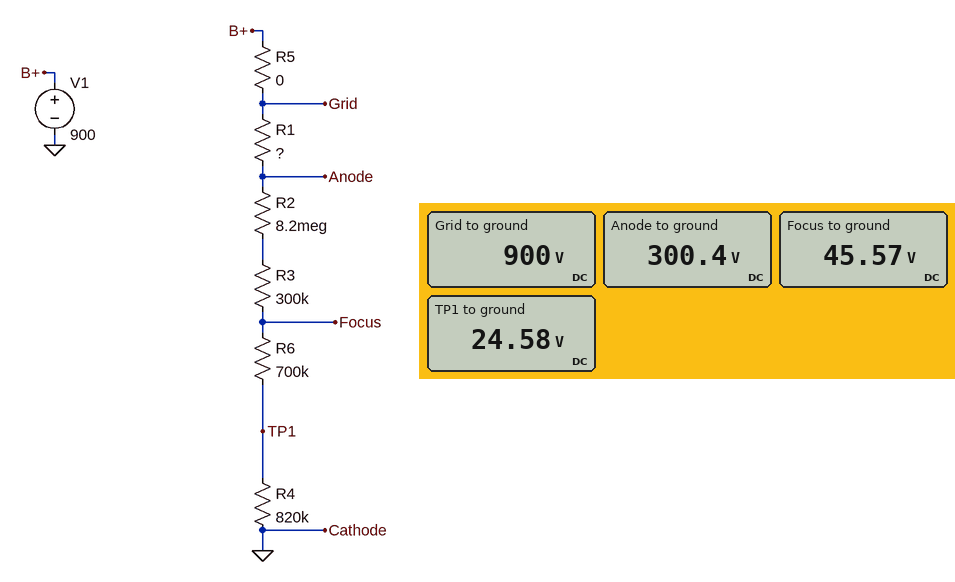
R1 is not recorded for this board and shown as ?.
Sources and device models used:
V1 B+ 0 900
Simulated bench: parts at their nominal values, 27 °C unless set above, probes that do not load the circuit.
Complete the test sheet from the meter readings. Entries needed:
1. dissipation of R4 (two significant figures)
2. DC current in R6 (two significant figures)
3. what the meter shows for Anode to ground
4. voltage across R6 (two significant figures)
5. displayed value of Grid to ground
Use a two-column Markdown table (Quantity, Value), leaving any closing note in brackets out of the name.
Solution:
| Quantity | Value |
|---|---|
| dissipation of R4 | 740 µW |
| DC current in R6 | 30 µA |
| what the meter shows for Anode to ground | 300.4 V |
| voltage across R6 | 21 V |
| displayed value of Grid to ground | 900 V |
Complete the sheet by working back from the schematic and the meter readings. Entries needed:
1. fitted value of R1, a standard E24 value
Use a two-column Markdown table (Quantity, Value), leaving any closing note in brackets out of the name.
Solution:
| Quantity | Value |
|---|---|
| fitted value of R1, a standard E24 value | 20 MΩ |
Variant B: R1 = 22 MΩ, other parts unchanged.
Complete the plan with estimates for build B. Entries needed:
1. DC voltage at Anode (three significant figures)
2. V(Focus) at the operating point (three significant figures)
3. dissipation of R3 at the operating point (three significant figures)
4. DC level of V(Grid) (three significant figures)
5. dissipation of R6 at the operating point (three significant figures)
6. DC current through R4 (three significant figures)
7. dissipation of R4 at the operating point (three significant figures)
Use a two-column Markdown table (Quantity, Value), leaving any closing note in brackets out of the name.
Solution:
| Quantity | Value |
|---|---|
| DC voltage at Anode | 282 V |
| V(Focus) at the operating point | 42.7 V |
| dissipation of R3 at the operating point | 237 µW |
| DC level of V(Grid) | 900 V |
| dissipation of R6 at the operating point | 553 µW |
| DC current through R4 | 28.1 µA |
| dissipation of R4 at the operating point | 648 µW |
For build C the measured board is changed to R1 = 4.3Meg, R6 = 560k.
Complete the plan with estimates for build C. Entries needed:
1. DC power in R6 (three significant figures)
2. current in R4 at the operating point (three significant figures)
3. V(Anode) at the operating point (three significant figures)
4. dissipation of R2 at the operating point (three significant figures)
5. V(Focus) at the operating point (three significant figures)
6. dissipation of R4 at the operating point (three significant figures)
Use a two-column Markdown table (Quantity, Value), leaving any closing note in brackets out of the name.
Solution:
| Quantity | Value |
|---|---|
| DC power in R6 | 2.26 mW |
| current in R4 at the operating point | 63.5 µA |
| V(Anode) at the operating point | 627 V |
| dissipation of R2 at the operating point | 33.0 mW |
| V(Focus) at the operating point | 87.6 V |
| dissipation of R4 at the operating point | 3.30 mW |
